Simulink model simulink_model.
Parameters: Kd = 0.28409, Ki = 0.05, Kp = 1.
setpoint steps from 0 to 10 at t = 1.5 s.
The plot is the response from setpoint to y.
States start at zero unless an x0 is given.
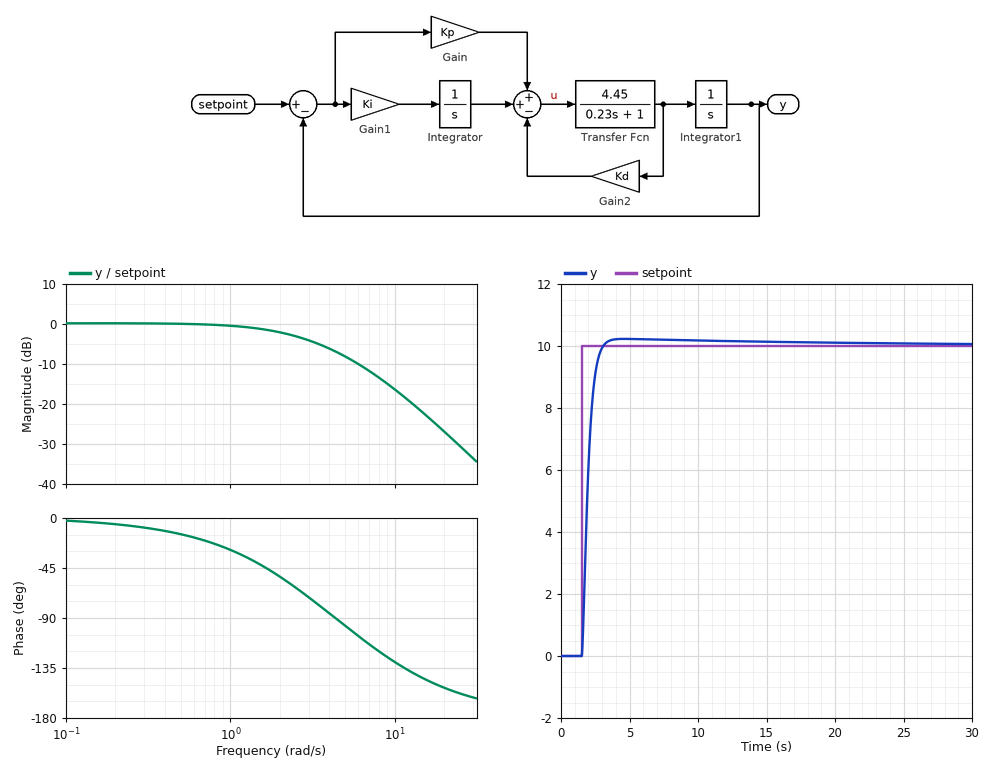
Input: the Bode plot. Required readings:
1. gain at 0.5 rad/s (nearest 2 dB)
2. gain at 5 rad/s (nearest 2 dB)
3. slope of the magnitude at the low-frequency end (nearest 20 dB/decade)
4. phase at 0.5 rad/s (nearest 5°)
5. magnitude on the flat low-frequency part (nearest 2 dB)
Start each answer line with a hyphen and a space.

- 0 dB
- -8 dB
- 0 dB/decade
- -15°
- 0 dB
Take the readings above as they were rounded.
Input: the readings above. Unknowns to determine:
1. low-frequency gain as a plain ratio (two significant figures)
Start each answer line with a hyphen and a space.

- 1.0
